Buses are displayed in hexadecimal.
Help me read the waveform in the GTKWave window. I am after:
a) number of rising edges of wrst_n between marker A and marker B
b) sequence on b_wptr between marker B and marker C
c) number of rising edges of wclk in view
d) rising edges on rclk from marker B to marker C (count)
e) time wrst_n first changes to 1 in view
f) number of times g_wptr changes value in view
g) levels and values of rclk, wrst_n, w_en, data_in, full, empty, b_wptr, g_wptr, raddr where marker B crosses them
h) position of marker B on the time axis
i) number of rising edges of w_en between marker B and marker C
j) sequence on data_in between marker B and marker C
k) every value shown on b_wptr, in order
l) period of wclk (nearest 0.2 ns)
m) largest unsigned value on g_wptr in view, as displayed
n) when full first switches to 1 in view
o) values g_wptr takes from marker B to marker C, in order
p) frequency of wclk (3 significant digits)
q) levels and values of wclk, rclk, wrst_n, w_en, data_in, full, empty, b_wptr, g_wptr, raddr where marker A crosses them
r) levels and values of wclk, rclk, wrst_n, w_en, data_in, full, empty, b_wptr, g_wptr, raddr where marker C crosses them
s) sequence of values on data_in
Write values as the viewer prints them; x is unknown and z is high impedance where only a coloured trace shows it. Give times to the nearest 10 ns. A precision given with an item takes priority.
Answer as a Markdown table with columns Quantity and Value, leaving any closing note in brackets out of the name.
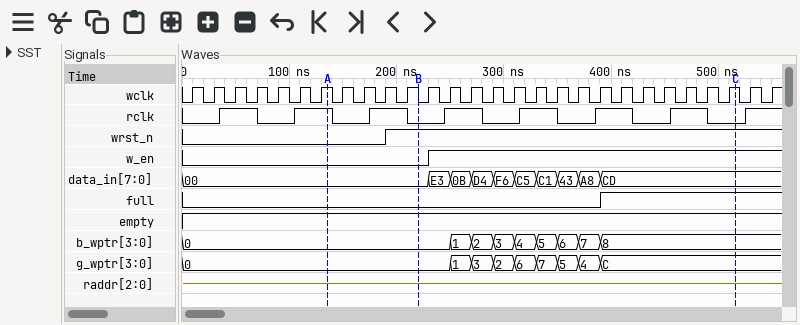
| Quantity | Value |
|---|---|
| number of rising edges of wrst_n between marker A and marker B | 1 |
| sequence on b_wptr between marker B and marker C | 0, 1, 2, 3, 4, 5, 6, 7, 8 |
| number of rising edges of wclk in view | 28 |
| rising edges on rclk from marker B to marker C | 4 |
| time wrst_n first changes to 1 in view | 190 ns |
| number of times g_wptr changes value in view | 8 |
| levels and values of rclk, wrst_n, w_en, data_in, full, empty, b_wptr, g_wptr, raddr where marker B crosses them | rclk=0, wrst_n=1, w_en=0, data_in=00, full=0, empty=1, b_wptr=0, g_wptr=0, raddr=z |
| position of marker B on the time axis | 220 ns |
| number of rising edges of w_en between marker B and marker C | 1 |
| sequence on data_in between marker B and marker C | 00, E3, 0B, D4, F6, C5, C1, 43, A8, CD |
| every value shown on b_wptr, in order | 0, 1, 2, 3, 4, 5, 6, 7, 8 |
| period of wclk | 20 ns |
| largest unsigned value on g_wptr in view, as displayed | C |
| when full first switches to 1 in view | 390 ns |
| values g_wptr takes from marker B to marker C, in order | 0, 1, 3, 2, 6, 7, 5, 4, C |
| frequency of wclk | 50.0 MHz |
| levels and values of wclk, rclk, wrst_n, w_en, data_in, full, empty, b_wptr, g_wptr, raddr where marker A crosses them | wclk=1, rclk=1, wrst_n=0, w_en=0, data_in=00, full=0, empty=1, b_wptr=0, g_wptr=0, raddr=z |
| levels and values of wclk, rclk, wrst_n, w_en, data_in, full, empty, b_wptr, g_wptr, raddr where marker C crosses them | wclk=1, rclk=0, wrst_n=1, w_en=1, data_in=CD, full=1, empty=1, b_wptr=8, g_wptr=C, raddr=z |
| sequence of values on data_in | 00, E3, 0B, D4, F6, C5, C1, 43, A8, CD |
